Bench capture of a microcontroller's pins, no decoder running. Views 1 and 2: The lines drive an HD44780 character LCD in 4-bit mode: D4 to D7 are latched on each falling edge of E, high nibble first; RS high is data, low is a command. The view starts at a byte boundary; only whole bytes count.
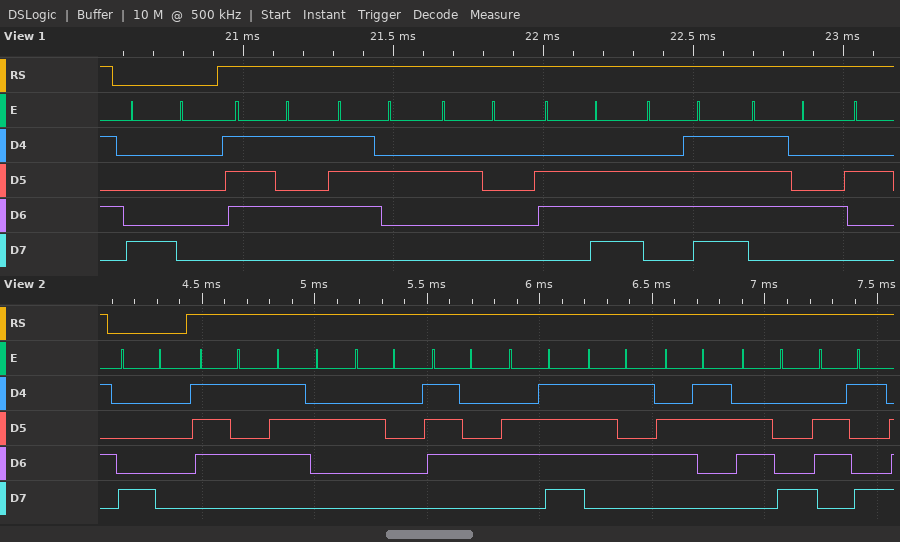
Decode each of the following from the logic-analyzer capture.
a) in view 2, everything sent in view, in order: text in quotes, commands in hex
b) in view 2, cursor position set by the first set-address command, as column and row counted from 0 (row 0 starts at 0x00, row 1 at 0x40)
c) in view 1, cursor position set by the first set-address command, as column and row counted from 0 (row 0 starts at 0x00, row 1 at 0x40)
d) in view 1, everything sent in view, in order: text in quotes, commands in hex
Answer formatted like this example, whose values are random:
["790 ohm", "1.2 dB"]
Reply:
["0x80 \"ur touchi\"", "column 0, row 0", "column 0, row 0", "0x80 \"ur not\""]
